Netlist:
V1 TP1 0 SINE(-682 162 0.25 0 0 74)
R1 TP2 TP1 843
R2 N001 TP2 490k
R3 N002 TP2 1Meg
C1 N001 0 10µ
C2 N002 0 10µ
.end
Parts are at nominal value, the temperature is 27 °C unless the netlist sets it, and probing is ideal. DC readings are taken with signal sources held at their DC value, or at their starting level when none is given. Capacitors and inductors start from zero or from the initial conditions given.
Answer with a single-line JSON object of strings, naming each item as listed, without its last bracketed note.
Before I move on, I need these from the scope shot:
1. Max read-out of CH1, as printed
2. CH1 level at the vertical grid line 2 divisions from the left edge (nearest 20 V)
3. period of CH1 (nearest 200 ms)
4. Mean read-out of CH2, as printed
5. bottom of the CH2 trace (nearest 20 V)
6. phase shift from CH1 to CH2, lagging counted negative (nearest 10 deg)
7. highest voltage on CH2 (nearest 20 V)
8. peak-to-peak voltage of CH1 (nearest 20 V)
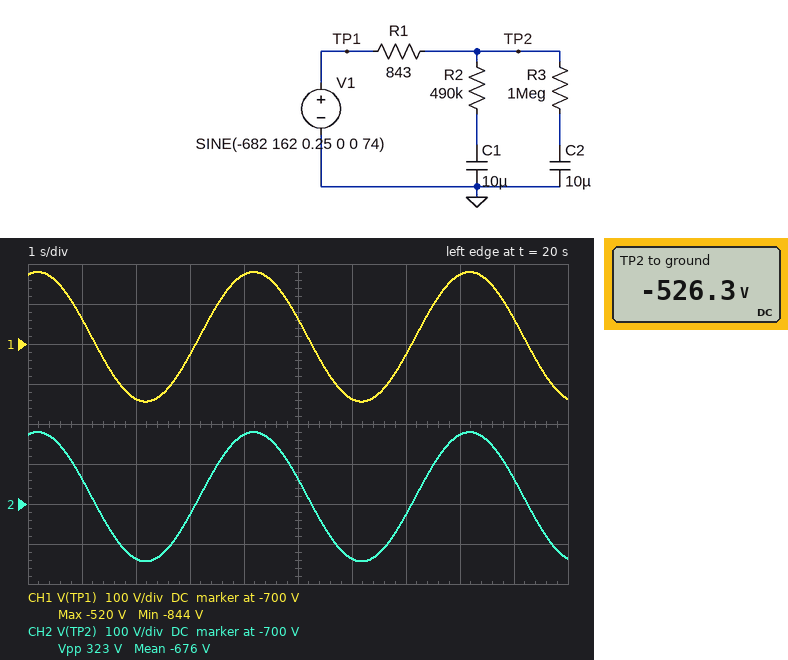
{"Max read-out of CH1, as printed": "-520 V", "CH1 level at the vertical grid line 2 divisions from the left edge": "-840 V", "period of CH1": "4.0 s", "Mean read-out of CH2, as printed": "-676 V", "bottom of the CH2 trace": "-840 V", "phase shift from CH1 to CH2, lagging counted negative": "0 deg", "highest voltage on CH2": "-520 V", "peak-to-peak voltage of CH1": "320 V"}
